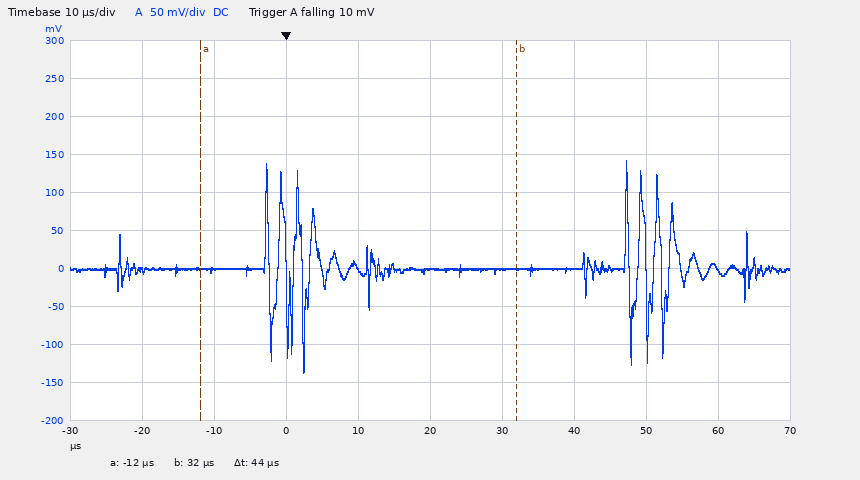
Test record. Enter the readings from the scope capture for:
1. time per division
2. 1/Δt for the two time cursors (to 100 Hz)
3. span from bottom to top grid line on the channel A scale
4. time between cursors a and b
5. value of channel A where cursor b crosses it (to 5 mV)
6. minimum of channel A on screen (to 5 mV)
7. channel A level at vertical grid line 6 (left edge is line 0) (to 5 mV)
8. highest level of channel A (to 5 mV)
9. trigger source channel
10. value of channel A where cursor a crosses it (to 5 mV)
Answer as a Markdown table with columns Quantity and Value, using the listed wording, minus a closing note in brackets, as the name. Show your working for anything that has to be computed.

| Quantity | Value |
|---|---|
| time per division | 10 µs |
| 1/Δt for the two time cursors | 1 / 44 µs ≈ 22.7 kHz |
| span from bottom to top grid line on the channel A scale | 500 mV |
| time between cursors a and b | 44 µs |
| value of channel A where cursor b crosses it | 0 mV |
| minimum of channel A on screen | -135 mV |
| channel A level at vertical grid line 6 (left edge is line 0) | 0 mV |
| highest level of channel A | 140 mV |
| trigger source channel | channel A |
| value of channel A where cursor a crosses it | 0 mV |
